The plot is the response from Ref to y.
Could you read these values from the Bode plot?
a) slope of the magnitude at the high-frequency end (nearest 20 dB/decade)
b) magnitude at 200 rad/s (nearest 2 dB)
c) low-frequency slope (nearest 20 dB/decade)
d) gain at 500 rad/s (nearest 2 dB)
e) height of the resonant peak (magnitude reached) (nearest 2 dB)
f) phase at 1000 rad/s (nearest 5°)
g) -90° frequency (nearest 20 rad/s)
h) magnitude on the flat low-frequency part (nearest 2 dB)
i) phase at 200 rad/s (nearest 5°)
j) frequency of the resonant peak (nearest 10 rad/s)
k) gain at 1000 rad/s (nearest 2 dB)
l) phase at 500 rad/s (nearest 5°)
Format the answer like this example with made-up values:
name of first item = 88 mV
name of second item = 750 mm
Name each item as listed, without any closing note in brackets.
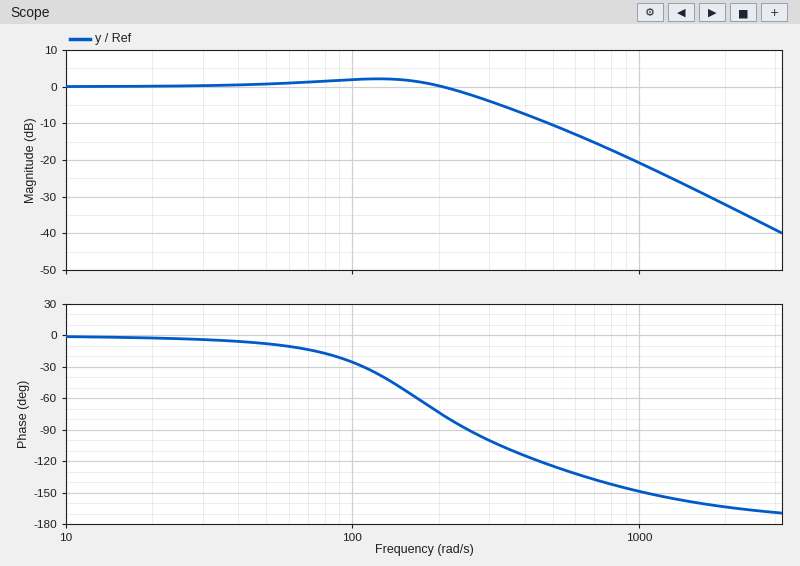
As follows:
slope of the magnitude at the high-frequency end = -40 dB/decade
magnitude at 200 rad/s = 0 dB
low-frequency slope = 0 dB/decade
gain at 500 rad/s = -10 dB
height of the resonant peak (magnitude reached) = 2 dB
phase at 1000 rad/s = -150°
-90° frequency = 260 rad/s
magnitude on the flat low-frequency part = 0 dB
phase at 200 rad/s = -75°
frequency of the resonant peak = 120 rad/s
gain at 1000 rad/s = -20 dB
phase at 500 rad/s = -125°
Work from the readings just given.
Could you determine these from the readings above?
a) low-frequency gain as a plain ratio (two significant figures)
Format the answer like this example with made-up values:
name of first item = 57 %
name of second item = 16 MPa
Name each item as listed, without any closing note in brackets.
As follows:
low-frequency gain as a plain ratio = 1.0
